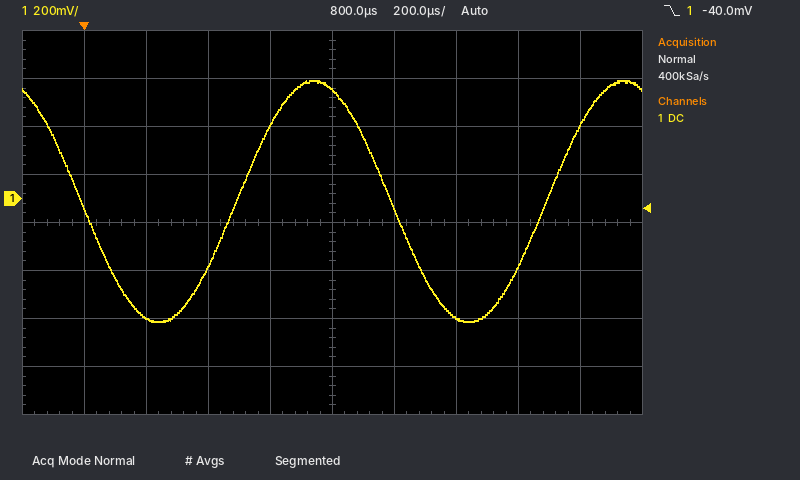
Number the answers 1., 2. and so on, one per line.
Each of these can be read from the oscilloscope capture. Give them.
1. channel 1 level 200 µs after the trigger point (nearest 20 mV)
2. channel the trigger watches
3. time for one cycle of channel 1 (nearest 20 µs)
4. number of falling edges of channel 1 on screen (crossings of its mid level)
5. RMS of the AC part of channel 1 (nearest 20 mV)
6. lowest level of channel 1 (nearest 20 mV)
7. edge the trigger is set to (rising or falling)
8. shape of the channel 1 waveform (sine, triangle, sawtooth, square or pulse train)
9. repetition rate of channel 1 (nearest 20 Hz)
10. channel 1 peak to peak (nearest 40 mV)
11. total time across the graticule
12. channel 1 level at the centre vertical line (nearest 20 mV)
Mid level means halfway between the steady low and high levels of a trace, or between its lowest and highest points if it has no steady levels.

1. -500 mV
2. channel 1
3. 1.00 ms
4. 2
5. 360 mV
6. -520 mV
7. falling
8. sine
9. 1.00 kHz
10. 1.00 V
11. 2 ms
12. 460 mV
